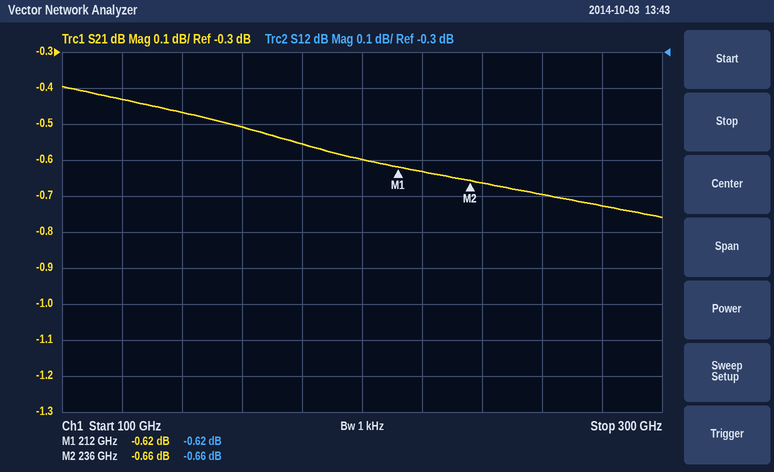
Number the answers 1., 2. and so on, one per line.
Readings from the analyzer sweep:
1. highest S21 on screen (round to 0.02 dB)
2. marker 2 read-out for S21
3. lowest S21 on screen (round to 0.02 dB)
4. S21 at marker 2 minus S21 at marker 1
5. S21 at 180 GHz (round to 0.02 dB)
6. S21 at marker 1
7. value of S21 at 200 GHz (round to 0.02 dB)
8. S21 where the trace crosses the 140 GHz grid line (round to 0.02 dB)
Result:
1. -0.40 dB
2. -0.66 dB
3. -0.76 dB
4. -0.04 dB
5. -0.56 dB
6. -0.62 dB
7. -0.60 dB
8. -0.46 dB
